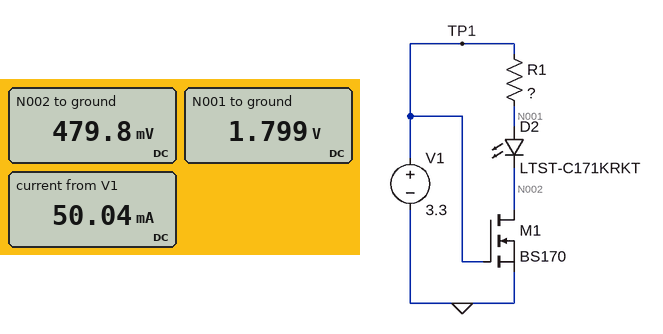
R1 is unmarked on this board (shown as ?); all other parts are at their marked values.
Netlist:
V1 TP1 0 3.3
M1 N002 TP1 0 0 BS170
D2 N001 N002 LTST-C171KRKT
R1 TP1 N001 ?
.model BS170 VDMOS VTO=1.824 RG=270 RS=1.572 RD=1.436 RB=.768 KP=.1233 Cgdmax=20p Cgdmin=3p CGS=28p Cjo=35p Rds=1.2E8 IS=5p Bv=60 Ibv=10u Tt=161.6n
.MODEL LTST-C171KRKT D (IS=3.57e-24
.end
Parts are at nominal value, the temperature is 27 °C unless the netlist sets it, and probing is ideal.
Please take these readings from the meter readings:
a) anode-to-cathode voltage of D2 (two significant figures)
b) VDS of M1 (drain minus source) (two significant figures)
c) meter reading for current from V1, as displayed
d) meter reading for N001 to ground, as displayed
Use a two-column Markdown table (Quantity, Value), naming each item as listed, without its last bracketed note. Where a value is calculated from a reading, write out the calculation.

| Quantity | Value |
|---|---|
| anode-to-cathode voltage of D2 | 1.799 V - 479.8 mV = 1.3 V |
| VDS of M1 (drain minus source) | 479.8 mV = 480 mV |
| meter reading for current from V1, as displayed | 50.04 mA |
| meter reading for N001 to ground, as displayed | 1.799 V |
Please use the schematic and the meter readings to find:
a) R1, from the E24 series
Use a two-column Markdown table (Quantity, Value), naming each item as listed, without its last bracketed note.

| Quantity | Value |
|---|---|
| R1, from the E24 series | 30 Ω |
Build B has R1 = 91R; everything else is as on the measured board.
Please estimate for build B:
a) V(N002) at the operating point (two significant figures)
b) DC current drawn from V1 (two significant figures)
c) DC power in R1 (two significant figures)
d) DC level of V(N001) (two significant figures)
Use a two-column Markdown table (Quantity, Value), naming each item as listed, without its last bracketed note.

| Quantity | Value |
|---|---|
| V(N002) at the operating point | 180 mV |
| DC current drawn from V1 | 20 mA |
| DC power in R1 | 37 mW |
| DC level of V(N001) | 1.5 V |
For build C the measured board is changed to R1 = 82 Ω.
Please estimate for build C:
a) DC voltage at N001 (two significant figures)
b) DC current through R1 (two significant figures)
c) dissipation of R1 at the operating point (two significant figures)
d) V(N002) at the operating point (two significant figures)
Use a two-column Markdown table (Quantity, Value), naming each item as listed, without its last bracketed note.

| Quantity | Value |
|---|---|
| DC voltage at N001 | 1.5 V |
| DC current through R1 | 22 mA |
| dissipation of R1 at the operating point | 40 mW |
| V(N002) at the operating point | 200 mV |
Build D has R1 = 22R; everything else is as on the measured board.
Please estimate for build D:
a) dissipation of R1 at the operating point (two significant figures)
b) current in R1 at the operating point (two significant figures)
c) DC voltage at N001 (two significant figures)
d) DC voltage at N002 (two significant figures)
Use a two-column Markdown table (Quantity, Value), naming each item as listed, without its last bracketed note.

| Quantity | Value |
|---|---|
| dissipation of R1 at the operating point | 84 mW |
| current in R1 at the operating point | 62 mA |
| DC voltage at N001 | 1.9 V |
| DC voltage at N002 | 620 mV |
